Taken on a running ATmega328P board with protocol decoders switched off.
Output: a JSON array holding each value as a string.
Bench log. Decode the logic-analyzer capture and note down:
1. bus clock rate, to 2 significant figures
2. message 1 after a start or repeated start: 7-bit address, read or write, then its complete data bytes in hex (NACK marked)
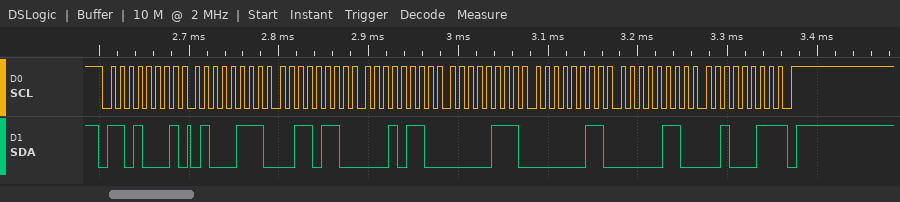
["100 kHz", "0x68 read: 47 36 16 07 03 06 23 NACK"]
